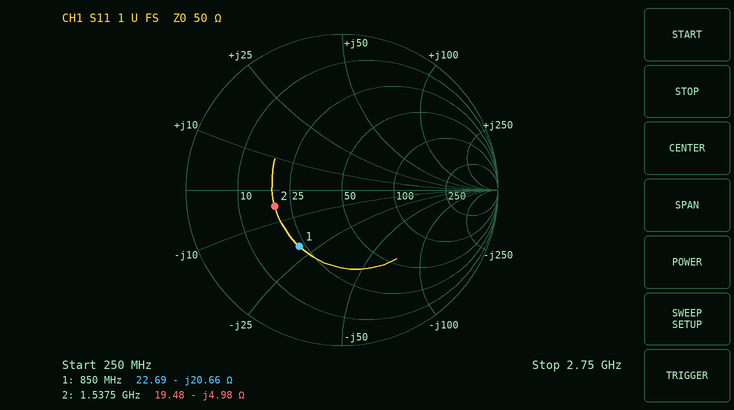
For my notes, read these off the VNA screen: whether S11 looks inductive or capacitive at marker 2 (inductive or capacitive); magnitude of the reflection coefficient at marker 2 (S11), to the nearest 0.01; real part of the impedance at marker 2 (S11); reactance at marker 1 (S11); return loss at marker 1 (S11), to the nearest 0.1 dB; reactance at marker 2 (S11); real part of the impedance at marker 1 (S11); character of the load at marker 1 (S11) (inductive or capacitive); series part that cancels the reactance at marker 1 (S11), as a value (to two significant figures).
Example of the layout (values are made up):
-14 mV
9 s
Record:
capacitive
0.44
19.48 Ω
-20.66 Ω
6.9 dB
-4.98 Ω
22.69 Ω
capacitive
3.9 nH
